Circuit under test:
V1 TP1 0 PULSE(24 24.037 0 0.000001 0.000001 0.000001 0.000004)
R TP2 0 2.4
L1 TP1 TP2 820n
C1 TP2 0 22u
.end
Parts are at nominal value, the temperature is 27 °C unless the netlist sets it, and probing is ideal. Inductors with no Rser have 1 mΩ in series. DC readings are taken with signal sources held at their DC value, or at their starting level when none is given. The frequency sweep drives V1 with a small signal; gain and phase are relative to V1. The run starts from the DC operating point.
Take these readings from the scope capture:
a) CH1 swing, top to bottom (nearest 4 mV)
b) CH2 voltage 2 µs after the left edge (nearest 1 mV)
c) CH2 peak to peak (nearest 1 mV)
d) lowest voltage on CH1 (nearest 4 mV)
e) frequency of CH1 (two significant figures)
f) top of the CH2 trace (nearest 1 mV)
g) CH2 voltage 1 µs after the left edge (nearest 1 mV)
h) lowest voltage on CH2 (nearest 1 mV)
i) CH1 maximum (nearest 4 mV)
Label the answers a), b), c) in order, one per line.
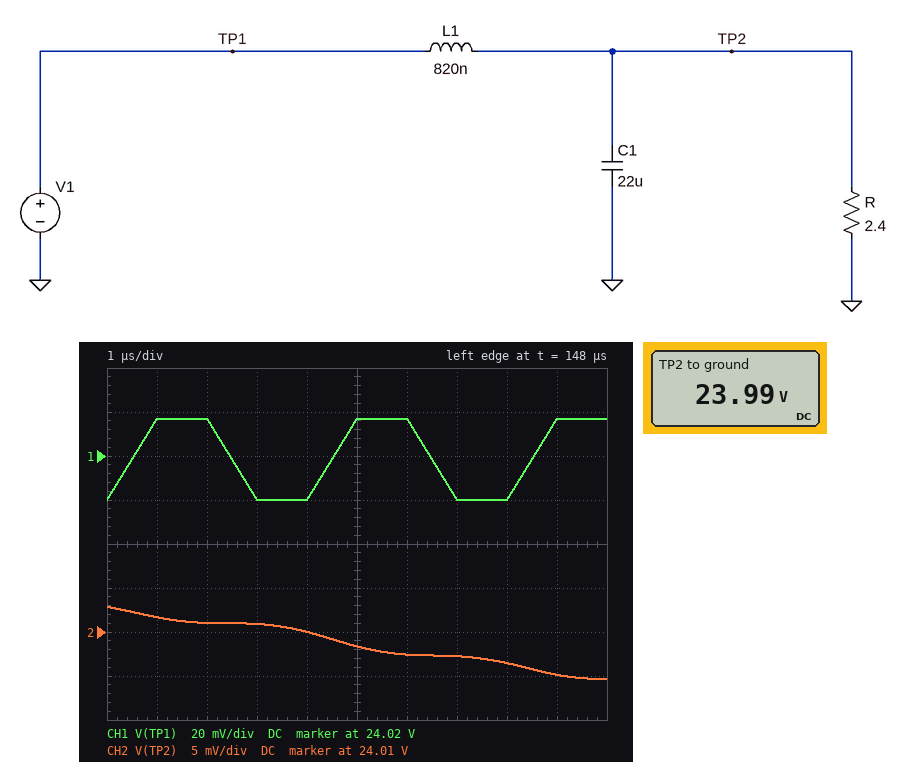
a) 36 mV
b) 24.011 V
c) 8 mV
d) 24.000 V
e) 250 kHz
f) 24.013 V
g) 24.012 V
h) 24.005 V
i) 24.036 V
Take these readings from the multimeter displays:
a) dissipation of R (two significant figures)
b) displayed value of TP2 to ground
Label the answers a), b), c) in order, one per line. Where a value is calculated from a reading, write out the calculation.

a) (23.99 V)^2 / 2.4 Ω = 240 W
b) 23.99 V
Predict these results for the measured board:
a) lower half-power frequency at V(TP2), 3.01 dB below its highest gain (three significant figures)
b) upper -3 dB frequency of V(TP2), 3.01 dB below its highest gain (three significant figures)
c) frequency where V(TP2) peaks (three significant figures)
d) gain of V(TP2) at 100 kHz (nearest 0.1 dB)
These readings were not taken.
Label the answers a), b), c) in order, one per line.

a) 35.8 kHz
b) 39.0 kHz
c) 37.4 kHz
d) -15.7 dB
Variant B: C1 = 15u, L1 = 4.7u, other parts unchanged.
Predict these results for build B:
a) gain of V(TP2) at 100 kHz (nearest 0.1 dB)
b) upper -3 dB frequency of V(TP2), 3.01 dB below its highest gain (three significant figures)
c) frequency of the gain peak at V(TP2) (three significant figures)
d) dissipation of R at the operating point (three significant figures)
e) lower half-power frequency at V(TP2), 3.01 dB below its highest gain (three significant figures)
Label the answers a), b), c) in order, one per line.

a) -28.6 dB
b) 20.8 kHz
c) 18.7 kHz
d) 240 W
e) 16.3 kHz
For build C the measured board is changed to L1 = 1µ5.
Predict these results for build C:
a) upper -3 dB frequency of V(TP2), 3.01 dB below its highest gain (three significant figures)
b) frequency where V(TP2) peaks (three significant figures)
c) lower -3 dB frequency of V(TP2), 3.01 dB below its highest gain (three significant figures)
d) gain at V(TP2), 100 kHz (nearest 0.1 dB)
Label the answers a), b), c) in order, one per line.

a) 29.1 kHz
b) 27.6 kHz
c) 26.0 kHz
d) -21.6 dB
